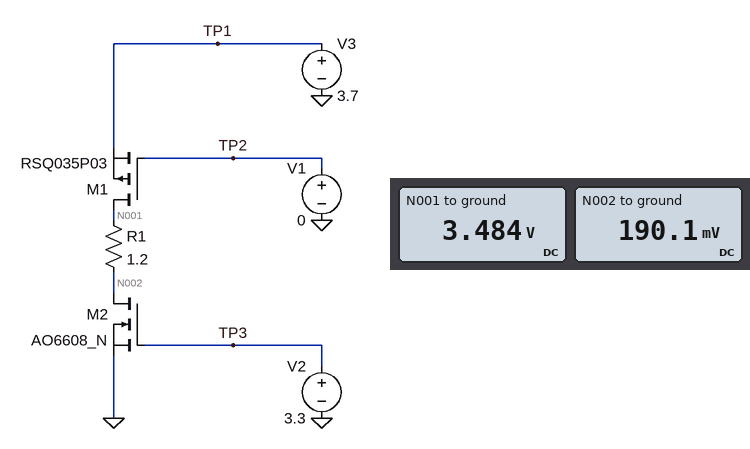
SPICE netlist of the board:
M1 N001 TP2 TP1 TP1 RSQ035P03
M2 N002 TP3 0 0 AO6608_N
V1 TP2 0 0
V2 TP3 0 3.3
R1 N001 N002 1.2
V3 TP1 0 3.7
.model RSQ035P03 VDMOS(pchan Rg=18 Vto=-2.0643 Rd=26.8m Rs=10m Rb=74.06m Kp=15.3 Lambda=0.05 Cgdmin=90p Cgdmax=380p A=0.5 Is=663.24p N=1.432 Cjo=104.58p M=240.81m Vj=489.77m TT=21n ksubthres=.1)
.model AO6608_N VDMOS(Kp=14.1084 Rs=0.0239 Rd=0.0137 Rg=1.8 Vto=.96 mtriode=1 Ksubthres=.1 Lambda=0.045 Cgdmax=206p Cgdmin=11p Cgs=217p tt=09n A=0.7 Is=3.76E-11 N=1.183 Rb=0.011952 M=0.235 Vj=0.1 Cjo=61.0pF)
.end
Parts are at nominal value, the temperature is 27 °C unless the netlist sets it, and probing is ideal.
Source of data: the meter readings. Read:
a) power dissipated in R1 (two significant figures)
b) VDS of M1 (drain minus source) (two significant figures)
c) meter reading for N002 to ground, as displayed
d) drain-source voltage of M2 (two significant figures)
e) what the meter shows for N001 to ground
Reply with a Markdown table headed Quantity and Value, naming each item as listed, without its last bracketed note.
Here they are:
| Quantity | Value |
|---|---|
| power dissipated in R1 | 9.0 W |
| VDS of M1 (drain minus source) | -220 mV |
| meter reading for N002 to ground, as displayed | 190.1 mV |
| drain-source voltage of M2 | 190 mV |
| what the meter shows for N001 to ground | 3.484 V |
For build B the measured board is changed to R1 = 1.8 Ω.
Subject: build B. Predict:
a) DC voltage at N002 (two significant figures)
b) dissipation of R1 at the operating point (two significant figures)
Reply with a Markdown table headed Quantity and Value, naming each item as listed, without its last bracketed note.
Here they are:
| Quantity | Value |
|---|---|
| DC voltage at N002 | 130 mV |
| dissipation of R1 at the operating point | 6.5 W |
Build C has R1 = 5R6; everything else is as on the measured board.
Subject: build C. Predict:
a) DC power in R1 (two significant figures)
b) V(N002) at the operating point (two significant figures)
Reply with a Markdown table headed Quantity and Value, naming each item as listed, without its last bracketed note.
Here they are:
| Quantity | Value |
|---|---|
| DC power in R1 | 2.3 W |
| V(N002) at the operating point | 44 mV |
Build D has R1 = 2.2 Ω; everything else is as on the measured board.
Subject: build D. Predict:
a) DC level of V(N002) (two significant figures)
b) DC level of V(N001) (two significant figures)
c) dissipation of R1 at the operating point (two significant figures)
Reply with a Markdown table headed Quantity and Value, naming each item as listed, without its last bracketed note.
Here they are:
| Quantity | Value |
|---|---|
| DC level of V(N002) | 110 mV |
| DC level of V(N001) | 3.6 V |
| dissipation of R1 at the operating point | 5.5 W |
